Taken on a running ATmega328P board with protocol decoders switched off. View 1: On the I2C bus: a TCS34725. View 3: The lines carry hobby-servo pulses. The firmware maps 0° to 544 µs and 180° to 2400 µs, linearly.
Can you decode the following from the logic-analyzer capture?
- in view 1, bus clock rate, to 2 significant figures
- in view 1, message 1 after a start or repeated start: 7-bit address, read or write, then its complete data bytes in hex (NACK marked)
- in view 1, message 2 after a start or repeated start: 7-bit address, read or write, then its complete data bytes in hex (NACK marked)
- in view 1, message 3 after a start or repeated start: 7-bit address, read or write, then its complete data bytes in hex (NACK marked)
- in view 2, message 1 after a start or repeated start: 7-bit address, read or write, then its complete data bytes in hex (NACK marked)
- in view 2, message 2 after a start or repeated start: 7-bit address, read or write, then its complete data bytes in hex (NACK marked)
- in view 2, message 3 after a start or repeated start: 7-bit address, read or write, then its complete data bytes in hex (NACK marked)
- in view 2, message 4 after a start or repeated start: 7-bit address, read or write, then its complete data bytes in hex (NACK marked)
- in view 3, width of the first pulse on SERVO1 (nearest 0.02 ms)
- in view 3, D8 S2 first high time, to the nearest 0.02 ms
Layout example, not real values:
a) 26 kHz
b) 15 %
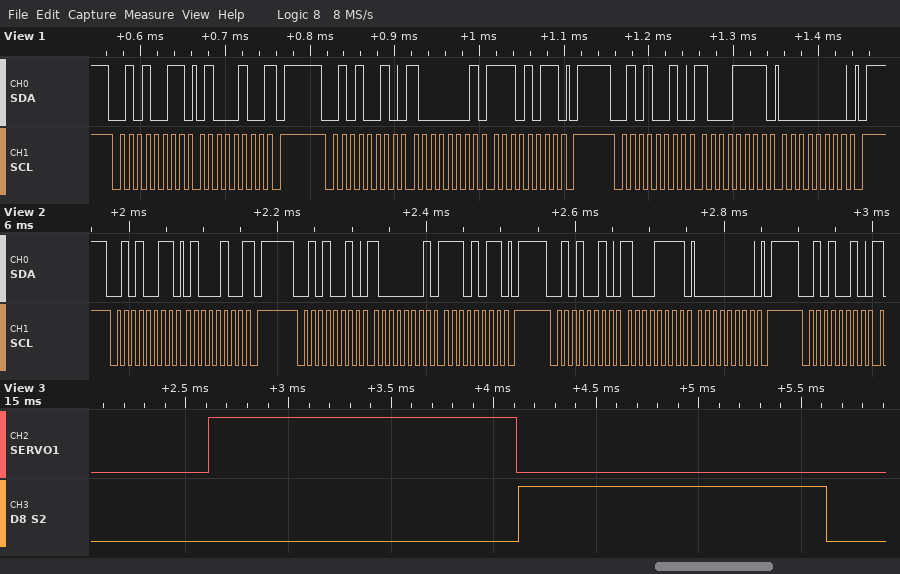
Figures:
a) 100 kHz
b) 0x29 read: 44 NACK
c) 0x29 write: 81 EB
d) 0x29 write: 8F 00
e) 0x29 read: 44 NACK
f) 0x29 write: 81 EB
g) 0x29 write: 8F 00
h) 0x29 write
i) 1.50 ms
j) 1.50 ms
